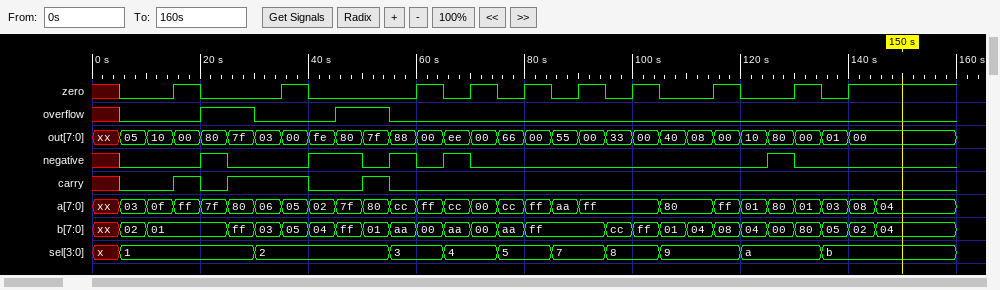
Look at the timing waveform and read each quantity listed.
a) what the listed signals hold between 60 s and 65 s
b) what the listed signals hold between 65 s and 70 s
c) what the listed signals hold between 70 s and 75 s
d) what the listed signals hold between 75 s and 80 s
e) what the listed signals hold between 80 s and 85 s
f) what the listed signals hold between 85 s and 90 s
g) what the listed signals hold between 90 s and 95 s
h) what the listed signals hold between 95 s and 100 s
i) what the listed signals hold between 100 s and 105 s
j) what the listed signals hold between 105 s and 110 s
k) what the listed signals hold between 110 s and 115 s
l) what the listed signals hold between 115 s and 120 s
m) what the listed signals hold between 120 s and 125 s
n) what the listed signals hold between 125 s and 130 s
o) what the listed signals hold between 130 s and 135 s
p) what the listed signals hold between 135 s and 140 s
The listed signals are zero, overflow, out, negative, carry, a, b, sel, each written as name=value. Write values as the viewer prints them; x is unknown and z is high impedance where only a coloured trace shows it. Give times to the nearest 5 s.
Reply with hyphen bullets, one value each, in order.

- zero=1, overflow=0, out=00, negative=0, carry=0, a=ff, b=00, sel=3
- zero=0, overflow=0, out=ee, negative=1, carry=0, a=cc, b=aa, sel=4
- zero=1, overflow=0, out=00, negative=0, carry=0, a=00, b=00, sel=4
- zero=0, overflow=0, out=66, negative=0, carry=0, a=cc, b=aa, sel=5
- zero=1, overflow=0, out=00, negative=0, carry=0, a=ff, b=ff, sel=5
- zero=0, overflow=0, out=55, negative=0, carry=0, a=aa, b=ff, sel=7
- zero=1, overflow=0, out=00, negative=0, carry=0, a=ff, b=ff, sel=7
- zero=0, overflow=0, out=33, negative=0, carry=0, a=ff, b=cc, sel=8
- zero=1, overflow=0, out=00, negative=0, carry=0, a=ff, b=ff, sel=8
- zero=0, overflow=0, out=40, negative=0, carry=0, a=80, b=01, sel=9
- zero=0, overflow=0, out=08, negative=0, carry=0, a=80, b=04, sel=9
- zero=1, overflow=0, out=00, negative=0, carry=0, a=ff, b=08, sel=9
- zero=0, overflow=0, out=10, negative=0, carry=0, a=01, b=04, sel=a
- zero=0, overflow=0, out=80, negative=1, carry=0, a=80, b=00, sel=a
- zero=1, overflow=0, out=00, negative=0, carry=0, a=01, b=80, sel=a
- zero=0, overflow=0, out=01, negative=0, carry=0, a=03, b=05, sel=b
